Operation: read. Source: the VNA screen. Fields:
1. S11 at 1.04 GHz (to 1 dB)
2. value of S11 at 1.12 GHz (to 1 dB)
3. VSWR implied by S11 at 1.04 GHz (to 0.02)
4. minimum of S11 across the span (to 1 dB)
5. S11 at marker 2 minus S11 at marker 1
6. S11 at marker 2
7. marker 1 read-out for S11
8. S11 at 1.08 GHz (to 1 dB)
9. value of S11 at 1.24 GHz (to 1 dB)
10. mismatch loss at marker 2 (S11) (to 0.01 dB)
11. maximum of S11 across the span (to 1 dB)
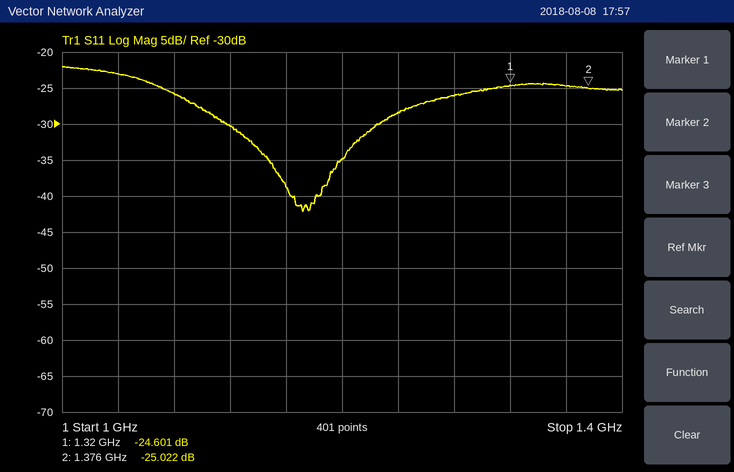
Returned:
-23 dB
-30 dB
1.16
-42 dB
-0.421 dB
-25.022 dB
-24.601 dB
-26 dB
-28 dB
0.01 dB
-22 dB
